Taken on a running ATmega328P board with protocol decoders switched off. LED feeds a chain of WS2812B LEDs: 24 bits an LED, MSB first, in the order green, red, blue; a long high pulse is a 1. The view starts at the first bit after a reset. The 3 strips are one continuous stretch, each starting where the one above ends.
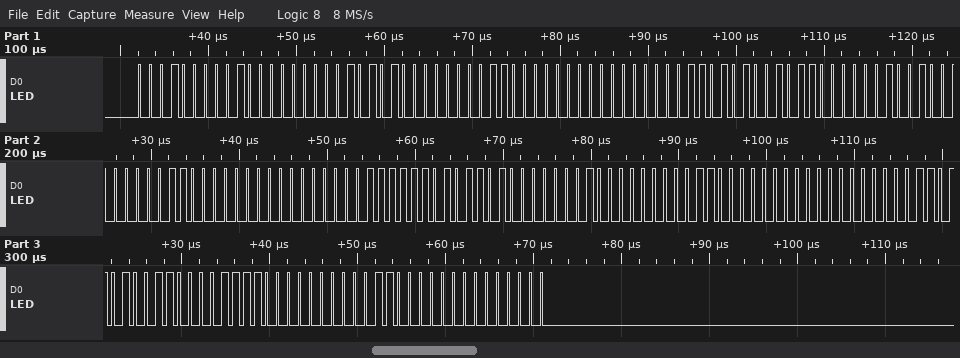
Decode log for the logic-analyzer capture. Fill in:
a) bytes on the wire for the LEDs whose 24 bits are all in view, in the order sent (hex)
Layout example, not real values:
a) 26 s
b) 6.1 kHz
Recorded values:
a) 10 40 15 00 C0 00 35 2C 09 00 C0 00 3F 5A 02 00 C0 00 0D 4C 3C 00 C0 00
